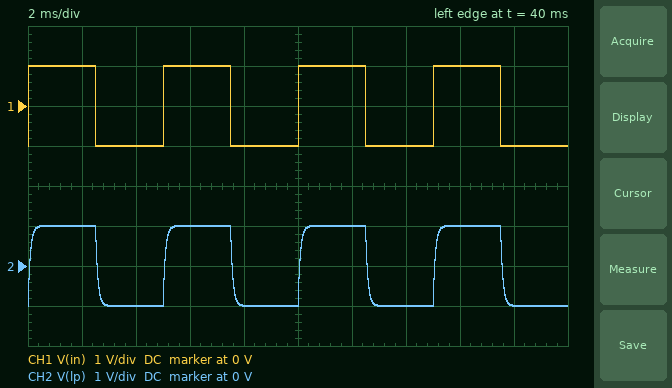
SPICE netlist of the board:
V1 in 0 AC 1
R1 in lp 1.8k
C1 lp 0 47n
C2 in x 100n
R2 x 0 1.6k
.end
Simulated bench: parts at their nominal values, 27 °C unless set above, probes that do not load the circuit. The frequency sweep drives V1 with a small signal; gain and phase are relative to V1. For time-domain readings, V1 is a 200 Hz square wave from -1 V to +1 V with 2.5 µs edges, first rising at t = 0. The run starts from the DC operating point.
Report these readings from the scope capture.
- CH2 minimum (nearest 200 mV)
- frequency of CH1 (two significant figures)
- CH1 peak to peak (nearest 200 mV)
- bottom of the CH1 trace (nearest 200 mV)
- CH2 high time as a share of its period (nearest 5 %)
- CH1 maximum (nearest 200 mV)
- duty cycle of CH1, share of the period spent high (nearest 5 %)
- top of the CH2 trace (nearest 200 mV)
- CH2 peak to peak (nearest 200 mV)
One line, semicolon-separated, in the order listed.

-1.0 V; 200 Hz; 2.0 V; -1.0 V; 50 %; 1.0 V; 50 %; 1.0 V; 2.0 V
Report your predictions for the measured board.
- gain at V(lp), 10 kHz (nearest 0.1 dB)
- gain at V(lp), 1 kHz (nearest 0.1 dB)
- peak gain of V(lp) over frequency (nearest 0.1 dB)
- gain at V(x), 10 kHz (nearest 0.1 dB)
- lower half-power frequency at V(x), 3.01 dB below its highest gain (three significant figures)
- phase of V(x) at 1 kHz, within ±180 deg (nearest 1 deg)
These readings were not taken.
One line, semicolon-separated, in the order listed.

-14.7 dB; -1.1 dB; 0 dB; 0 dB; 995 Hz; 45 deg
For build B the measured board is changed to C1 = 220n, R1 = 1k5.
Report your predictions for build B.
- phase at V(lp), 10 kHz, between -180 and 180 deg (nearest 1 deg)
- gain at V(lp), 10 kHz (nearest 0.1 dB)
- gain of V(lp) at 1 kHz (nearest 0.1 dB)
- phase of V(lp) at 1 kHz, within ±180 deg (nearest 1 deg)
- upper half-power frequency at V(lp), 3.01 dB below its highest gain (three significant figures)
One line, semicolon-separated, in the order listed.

-87 deg; -26.3 dB; -7.2 dB; -64 deg; 482 Hz
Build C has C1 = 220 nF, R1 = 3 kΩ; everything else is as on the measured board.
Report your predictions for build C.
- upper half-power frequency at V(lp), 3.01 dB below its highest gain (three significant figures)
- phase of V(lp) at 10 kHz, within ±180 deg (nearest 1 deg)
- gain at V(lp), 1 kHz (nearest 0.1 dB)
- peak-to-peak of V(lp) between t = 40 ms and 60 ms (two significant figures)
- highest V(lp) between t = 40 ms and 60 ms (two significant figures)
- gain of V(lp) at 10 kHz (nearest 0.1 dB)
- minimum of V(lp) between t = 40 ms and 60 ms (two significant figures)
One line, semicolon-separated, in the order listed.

241 Hz; -89 deg; -12.6 dB; 1.9 V; 960 mV; -32.4 dB; -960 mV
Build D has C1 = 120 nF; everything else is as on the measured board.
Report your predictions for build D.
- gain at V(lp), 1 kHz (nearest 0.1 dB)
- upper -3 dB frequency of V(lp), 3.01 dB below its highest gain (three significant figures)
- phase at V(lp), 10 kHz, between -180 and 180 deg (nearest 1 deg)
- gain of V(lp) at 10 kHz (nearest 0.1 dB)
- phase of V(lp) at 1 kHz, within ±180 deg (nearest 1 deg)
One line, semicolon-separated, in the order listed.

-4.5 dB; 737 Hz; -86 deg; -22.7 dB; -54 deg
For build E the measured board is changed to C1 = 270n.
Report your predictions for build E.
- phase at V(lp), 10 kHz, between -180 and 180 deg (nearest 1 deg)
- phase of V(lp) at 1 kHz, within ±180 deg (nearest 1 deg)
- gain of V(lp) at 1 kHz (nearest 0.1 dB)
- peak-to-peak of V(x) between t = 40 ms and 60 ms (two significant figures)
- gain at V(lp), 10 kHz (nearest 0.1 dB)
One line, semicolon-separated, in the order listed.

-88 deg; -72 deg; -10.1 dB; 4.0 V; -29.7 dB
